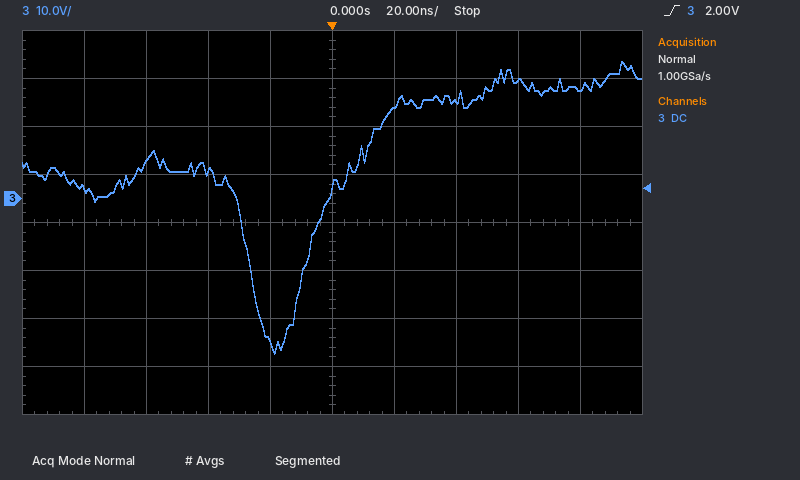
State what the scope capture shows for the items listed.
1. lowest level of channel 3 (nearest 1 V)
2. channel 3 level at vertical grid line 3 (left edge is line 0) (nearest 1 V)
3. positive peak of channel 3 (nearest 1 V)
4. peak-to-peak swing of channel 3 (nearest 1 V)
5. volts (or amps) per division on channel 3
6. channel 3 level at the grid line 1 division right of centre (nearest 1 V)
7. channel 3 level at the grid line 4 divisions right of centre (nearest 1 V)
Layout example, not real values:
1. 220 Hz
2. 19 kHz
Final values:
1. -32 V
2. 6 V
3. 29 V
4. 61 V
5. 10 V
6. 19 V
7. 23 V
